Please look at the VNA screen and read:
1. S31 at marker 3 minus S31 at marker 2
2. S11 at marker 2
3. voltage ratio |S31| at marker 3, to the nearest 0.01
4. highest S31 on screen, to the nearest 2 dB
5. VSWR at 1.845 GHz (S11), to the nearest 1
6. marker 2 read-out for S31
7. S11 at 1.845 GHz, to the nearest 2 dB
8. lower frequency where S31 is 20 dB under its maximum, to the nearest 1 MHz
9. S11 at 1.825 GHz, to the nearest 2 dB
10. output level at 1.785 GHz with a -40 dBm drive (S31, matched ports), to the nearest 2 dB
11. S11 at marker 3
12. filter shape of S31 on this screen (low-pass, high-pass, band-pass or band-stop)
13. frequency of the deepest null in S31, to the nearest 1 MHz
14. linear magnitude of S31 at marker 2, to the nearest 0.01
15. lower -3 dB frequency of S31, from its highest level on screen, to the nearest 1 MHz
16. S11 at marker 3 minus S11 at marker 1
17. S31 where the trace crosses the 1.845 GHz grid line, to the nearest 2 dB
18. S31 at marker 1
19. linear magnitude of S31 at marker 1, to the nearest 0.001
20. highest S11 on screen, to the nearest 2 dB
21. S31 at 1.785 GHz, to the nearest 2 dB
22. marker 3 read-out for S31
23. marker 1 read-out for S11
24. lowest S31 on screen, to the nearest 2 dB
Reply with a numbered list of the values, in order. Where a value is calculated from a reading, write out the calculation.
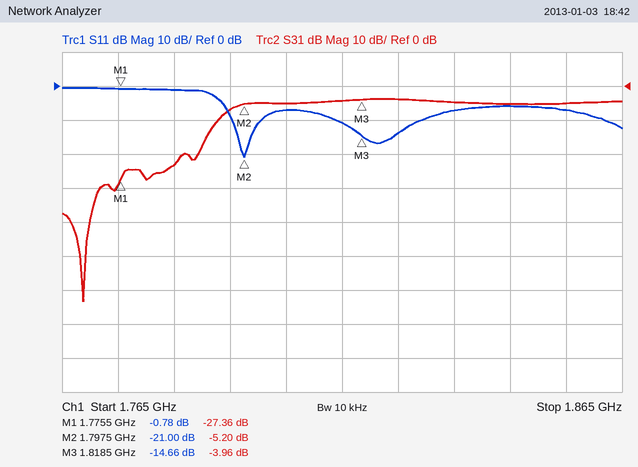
1. -3.96 − (-5.2) = 1.24 dB
2. -21.00 dB
3. 10^(-3.96/20) ≈ 0.63
4. -4 dB
5. |Γ| = 10^(-6/20) = 0.5012; VSWR = (1 + 0.5012)/(1 − 0.5012) ≈ 3
6. -5.20 dB
7. -6 dB
8. 1.784 GHz
9. -14 dB
10. -40 dBm + (-24 dB) = -64 dBm
11. -14.66 dB
12. high-pass
13. 1.769 GHz
14. 10^(-5.2/20) ≈ 0.55
15. 1.795 GHz
16. -14.66 − (-0.78) = -13.88 dB
17. -6 dB
18. -27.36 dB
19. 10^(-27.36/20) ≈ 0.043
20. 0 dB
21. -24 dB
22. -3.96 dB
23. -0.78 dB
24. -64 dB
